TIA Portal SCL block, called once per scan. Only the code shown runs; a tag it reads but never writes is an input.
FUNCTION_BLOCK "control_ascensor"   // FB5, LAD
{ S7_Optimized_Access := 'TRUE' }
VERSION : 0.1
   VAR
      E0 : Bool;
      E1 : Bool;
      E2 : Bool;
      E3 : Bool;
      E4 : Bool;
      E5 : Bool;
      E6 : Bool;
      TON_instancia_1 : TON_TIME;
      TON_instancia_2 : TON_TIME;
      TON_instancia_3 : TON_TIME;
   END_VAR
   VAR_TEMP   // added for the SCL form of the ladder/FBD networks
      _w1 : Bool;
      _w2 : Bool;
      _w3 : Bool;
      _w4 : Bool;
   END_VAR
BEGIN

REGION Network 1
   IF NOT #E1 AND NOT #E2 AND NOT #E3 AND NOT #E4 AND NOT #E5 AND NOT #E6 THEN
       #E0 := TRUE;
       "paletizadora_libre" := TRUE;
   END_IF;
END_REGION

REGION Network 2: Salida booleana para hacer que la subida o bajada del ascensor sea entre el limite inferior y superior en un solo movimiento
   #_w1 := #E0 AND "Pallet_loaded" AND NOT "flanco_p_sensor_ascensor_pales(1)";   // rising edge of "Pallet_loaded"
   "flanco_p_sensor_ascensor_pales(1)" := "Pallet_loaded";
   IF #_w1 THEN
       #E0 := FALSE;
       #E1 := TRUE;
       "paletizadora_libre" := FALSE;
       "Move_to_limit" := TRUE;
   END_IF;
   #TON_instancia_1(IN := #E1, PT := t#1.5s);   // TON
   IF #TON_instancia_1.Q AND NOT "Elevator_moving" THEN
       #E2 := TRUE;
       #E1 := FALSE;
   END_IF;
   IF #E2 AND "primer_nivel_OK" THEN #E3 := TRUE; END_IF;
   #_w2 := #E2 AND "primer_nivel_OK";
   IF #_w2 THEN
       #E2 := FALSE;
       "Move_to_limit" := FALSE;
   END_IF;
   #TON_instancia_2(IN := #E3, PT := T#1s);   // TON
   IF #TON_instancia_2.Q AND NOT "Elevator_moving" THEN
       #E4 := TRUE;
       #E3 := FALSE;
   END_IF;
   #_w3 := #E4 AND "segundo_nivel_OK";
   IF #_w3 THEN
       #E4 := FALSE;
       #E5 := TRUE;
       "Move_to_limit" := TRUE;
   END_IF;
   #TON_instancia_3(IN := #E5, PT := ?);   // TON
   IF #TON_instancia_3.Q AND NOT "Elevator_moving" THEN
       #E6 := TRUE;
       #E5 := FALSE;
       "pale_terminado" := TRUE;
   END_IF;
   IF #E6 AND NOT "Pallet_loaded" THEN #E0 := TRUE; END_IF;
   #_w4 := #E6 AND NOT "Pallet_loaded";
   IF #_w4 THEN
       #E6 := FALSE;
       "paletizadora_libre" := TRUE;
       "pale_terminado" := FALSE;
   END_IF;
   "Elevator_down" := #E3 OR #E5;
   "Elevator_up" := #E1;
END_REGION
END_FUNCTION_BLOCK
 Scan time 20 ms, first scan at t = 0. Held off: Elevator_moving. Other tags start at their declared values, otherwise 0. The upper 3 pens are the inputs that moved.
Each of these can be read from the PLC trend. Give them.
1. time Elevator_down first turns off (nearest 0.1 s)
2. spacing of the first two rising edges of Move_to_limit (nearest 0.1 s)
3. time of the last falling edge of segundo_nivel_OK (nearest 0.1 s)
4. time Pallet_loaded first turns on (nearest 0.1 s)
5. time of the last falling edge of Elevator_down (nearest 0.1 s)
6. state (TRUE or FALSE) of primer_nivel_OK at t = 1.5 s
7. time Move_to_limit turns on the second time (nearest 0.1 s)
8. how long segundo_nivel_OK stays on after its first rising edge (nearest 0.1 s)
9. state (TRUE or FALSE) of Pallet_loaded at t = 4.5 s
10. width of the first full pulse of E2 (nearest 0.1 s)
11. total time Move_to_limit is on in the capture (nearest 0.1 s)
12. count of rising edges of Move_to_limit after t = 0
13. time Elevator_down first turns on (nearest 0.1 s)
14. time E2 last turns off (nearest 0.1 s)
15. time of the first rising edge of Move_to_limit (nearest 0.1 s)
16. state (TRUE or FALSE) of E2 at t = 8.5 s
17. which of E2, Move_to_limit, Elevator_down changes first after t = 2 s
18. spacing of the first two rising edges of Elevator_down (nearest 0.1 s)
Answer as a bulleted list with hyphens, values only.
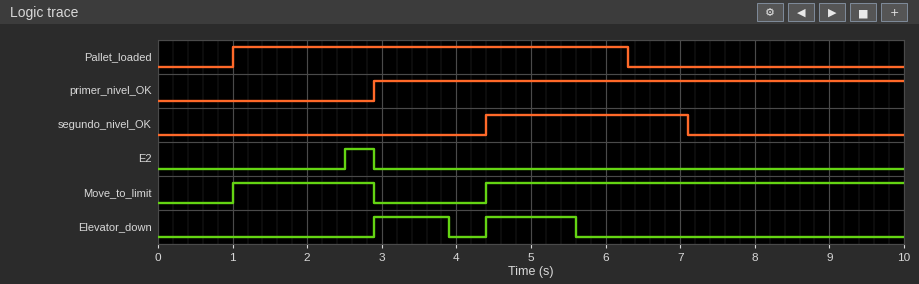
- 3.9 s
- 3.4 s
- 7.1 s
- 1.0 s
- 5.6 s
- FALSE
- 4.4 s
- 2.7 s
- TRUE
- 0.4 s
- 7.5 s
- 2
- 2.9 s
- 2.9 s
- 1.0 s
- FALSE
- E2
- 1.5 s
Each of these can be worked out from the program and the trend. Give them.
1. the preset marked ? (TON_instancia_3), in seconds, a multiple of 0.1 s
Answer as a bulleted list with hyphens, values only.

- 1.2 s
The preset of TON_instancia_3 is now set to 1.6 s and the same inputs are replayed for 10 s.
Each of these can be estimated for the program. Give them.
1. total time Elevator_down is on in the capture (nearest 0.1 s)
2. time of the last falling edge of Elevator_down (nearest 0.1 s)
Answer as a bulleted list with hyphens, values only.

- 2.6 s
- 6.0 s
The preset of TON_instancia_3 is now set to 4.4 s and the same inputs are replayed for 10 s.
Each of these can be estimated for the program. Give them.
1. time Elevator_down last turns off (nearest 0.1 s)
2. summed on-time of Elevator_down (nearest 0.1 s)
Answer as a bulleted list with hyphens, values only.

- 8.8 s
- 5.4 s
